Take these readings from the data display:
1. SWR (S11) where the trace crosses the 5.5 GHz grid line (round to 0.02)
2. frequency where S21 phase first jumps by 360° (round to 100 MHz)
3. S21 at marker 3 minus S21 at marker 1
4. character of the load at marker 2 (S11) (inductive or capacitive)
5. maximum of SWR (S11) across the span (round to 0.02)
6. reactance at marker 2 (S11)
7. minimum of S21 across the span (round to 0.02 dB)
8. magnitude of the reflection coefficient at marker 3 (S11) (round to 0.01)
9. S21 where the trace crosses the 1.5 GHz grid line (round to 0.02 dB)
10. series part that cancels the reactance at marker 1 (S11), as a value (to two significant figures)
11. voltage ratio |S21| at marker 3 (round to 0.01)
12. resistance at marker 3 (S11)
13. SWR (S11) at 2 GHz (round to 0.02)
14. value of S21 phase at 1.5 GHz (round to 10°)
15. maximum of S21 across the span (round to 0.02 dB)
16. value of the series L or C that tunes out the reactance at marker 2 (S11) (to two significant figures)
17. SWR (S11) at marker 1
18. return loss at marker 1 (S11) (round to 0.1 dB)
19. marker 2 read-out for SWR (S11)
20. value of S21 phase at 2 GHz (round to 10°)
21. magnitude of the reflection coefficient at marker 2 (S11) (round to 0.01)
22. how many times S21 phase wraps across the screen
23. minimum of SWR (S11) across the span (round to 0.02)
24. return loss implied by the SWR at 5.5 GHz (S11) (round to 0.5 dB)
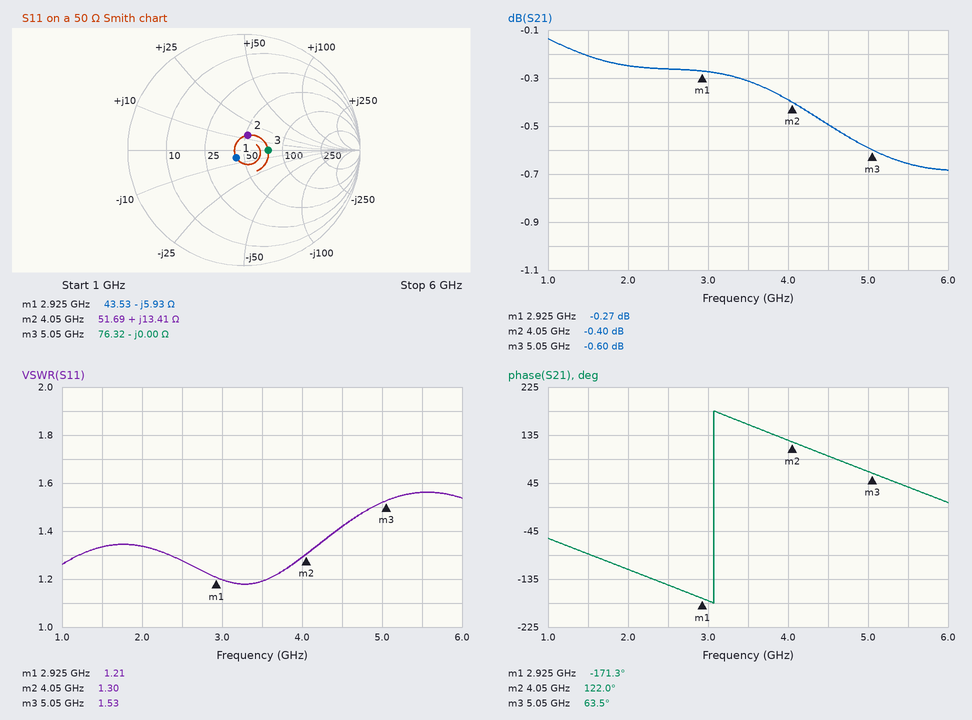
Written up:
1.56
3.1 GHz
-0.33 dB
inductive
1.56
+13.41 Ω
-0.68 dB
0.21
-0.20 dB
320 pH
0.93
76.32 Ω
1.34
-90°
-0.14 dB
2.9 pF
1.21
20.6 dB
1.30
-120°
0.13
1
1.18
13.0 dB
